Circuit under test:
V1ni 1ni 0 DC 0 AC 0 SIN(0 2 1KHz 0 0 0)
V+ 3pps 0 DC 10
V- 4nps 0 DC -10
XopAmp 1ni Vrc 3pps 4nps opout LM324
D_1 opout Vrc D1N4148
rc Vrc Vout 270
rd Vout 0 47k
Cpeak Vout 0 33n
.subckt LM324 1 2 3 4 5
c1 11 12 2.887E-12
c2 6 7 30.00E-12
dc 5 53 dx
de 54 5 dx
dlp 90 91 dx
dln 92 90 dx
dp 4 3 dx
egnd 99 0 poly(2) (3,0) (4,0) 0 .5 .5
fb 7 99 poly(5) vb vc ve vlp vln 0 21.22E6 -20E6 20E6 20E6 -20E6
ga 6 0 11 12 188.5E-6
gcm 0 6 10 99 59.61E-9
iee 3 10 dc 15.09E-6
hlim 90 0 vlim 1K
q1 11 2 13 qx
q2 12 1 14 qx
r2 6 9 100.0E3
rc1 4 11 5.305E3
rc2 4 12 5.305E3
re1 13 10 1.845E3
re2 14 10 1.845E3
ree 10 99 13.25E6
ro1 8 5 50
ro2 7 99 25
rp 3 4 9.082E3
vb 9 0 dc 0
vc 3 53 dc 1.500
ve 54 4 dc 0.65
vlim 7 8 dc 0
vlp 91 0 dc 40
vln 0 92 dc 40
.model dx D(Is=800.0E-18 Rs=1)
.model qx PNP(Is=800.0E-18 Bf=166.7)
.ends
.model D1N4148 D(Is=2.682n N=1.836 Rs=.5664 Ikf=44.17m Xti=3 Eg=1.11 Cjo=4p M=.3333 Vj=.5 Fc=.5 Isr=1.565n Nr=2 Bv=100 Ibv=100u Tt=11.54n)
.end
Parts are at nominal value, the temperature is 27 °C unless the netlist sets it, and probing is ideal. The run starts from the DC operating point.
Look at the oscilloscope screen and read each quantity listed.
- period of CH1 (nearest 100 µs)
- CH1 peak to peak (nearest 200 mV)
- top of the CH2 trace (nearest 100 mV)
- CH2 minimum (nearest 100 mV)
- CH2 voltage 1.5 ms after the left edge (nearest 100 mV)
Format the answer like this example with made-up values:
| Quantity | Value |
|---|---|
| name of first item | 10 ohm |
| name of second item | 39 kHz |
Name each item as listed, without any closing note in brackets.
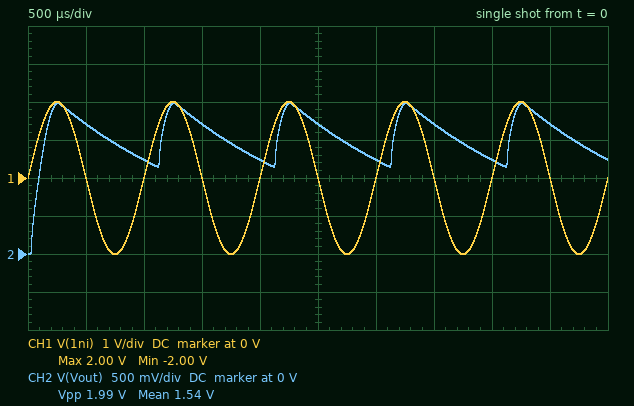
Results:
| Quantity | Value |
|---|---|
| period of CH1 | 1.0 ms |
| CH1 peak to peak | 4.0 V |
| top of the CH2 trace | 2.0 V |
| CH2 minimum | 0 V |
| CH2 voltage 1.5 ms after the left edge | 1.7 V |
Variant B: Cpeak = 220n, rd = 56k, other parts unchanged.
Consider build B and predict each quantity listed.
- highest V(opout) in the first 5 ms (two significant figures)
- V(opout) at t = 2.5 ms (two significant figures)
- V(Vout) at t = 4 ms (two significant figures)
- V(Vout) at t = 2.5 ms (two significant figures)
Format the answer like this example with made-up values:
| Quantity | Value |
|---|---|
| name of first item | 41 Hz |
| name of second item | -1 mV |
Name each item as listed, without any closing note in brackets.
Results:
| Quantity | Value |
|---|---|
| highest V(opout) in the first 5 ms | 2.6 V |
| V(opout) at t = 2.5 ms | -10 V |
| V(Vout) at t = 4 ms | 1.8 V |
| V(Vout) at t = 2.5 ms | 1.9 V |
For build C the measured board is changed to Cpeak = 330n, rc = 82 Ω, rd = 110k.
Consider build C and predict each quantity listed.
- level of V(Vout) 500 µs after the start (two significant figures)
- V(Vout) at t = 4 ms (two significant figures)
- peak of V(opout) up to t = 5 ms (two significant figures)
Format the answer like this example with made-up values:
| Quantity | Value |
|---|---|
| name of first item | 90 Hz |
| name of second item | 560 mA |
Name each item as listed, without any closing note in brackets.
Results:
| Quantity | Value |
|---|---|
| level of V(Vout) 500 µs after the start | 2.0 V |
| V(Vout) at t = 4 ms | 1.9 V |
| peak of V(opout) up to t = 5 ms | 2.6 V |
